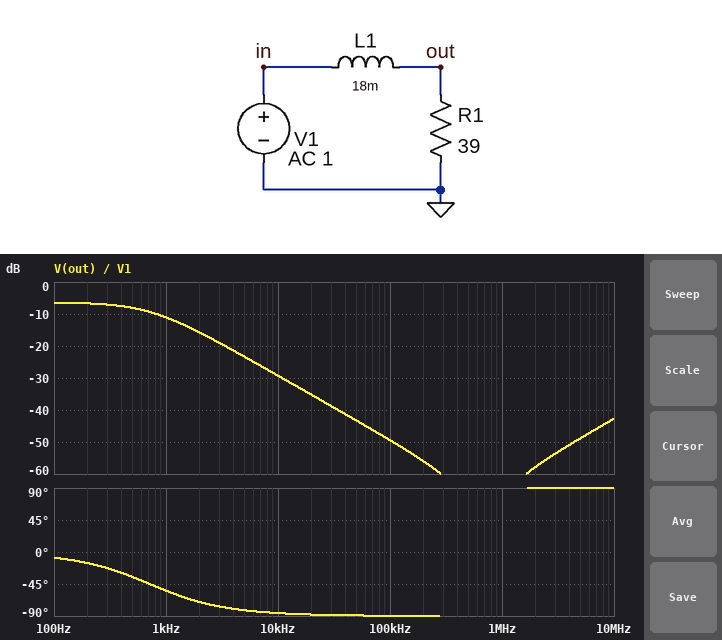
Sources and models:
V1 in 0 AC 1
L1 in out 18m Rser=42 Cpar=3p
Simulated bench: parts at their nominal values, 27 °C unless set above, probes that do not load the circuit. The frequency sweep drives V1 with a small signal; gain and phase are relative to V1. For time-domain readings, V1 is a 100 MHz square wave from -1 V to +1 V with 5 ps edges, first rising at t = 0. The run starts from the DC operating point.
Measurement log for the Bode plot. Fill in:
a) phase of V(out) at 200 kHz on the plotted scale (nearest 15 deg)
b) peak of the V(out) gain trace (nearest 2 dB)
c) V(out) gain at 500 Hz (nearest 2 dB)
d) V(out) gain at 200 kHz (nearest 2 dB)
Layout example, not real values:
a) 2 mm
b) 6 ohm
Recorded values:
a) -90 deg
b) -6 dB
c) -8 dB
d) -56 dB
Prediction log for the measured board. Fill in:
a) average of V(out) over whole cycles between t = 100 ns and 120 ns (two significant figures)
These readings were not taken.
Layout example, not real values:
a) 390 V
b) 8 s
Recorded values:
a) -480 mV
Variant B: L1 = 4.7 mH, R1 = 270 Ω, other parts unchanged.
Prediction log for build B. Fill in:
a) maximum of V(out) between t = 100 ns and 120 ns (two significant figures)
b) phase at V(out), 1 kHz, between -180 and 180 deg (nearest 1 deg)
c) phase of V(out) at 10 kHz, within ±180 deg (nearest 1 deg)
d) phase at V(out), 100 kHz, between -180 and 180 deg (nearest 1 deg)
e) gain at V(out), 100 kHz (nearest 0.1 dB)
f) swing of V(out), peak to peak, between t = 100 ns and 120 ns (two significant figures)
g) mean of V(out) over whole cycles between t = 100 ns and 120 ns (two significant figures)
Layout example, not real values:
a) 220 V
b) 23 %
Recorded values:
a) 1.1 V
b) -5 deg
c) -43 deg
d) -84 deg
e) -20.9 dB
f) 4.0 V
g) -860 mV
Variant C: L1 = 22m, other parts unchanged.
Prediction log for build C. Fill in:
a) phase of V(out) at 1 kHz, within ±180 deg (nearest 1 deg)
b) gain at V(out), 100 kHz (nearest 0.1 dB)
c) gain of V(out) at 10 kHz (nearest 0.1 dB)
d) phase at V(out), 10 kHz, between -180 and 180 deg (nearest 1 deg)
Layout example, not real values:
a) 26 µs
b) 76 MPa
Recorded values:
a) -60 deg
b) -51.2 dB
c) -31.0 dB
d) -87 deg
